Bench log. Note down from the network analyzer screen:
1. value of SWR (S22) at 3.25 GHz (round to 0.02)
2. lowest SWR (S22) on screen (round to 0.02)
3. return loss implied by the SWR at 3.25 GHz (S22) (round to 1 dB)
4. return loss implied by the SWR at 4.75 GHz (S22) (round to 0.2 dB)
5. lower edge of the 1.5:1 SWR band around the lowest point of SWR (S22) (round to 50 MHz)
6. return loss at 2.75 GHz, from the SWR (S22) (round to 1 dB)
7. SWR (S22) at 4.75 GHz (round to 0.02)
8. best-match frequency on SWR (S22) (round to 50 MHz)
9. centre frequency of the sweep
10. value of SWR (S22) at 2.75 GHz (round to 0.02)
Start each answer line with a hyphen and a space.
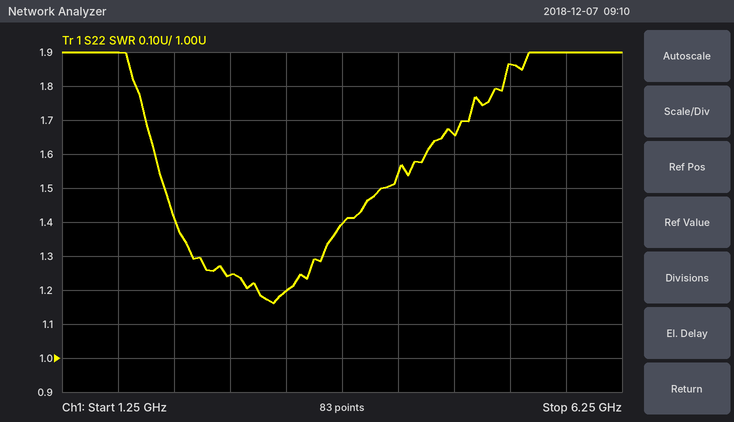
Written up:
- 1.20
- 1.16
- 21 dB
- 12.2 dB
- 2.15 GHz
- 19 dB
- 1.66
- 3.15 GHz
- 3.75 GHz
- 1.24
